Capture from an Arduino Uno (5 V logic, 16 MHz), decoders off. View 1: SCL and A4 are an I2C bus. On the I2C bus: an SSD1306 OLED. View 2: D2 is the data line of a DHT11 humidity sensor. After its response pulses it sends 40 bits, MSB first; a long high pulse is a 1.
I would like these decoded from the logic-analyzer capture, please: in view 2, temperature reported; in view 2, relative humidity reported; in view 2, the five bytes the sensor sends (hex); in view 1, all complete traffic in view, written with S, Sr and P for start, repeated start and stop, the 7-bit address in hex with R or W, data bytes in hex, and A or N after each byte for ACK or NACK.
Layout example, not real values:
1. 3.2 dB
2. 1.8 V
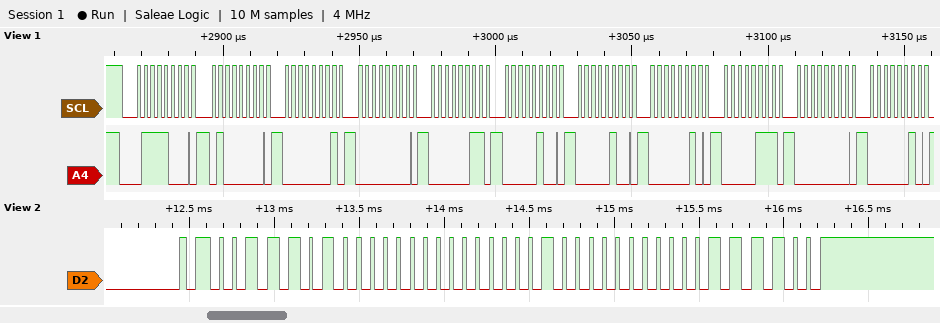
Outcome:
1. 2.0 °C
2. 58 %
3. 3A 00 02 00 3C
4. S 3CW A 40 A 01 A 00 A 03 A 04 A 04 A 02 A 07 A 00 A 02 A
